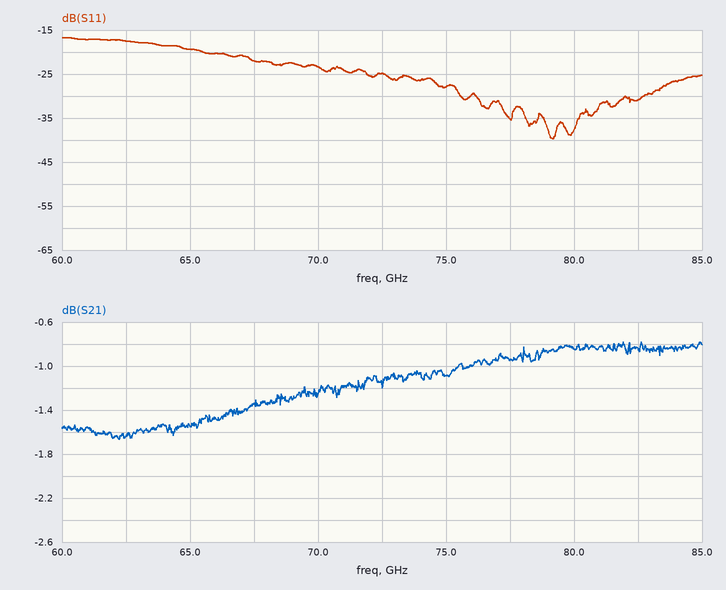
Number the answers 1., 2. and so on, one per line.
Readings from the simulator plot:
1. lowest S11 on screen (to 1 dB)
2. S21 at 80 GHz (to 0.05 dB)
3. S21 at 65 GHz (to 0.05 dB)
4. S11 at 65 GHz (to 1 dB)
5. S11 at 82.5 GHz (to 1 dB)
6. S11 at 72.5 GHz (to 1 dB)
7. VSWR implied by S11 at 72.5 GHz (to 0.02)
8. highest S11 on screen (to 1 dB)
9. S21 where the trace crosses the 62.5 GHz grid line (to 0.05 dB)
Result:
1. -40 dB
2. -0.85 dB
3. -1.55 dB
4. -19 dB
5. -31 dB
6. -25 dB
7. 1.12
8. -17 dB
9. -1.65 dB
